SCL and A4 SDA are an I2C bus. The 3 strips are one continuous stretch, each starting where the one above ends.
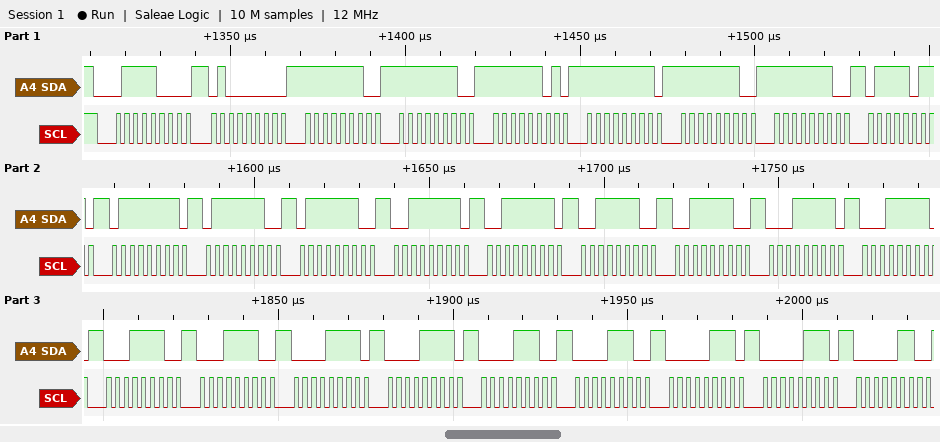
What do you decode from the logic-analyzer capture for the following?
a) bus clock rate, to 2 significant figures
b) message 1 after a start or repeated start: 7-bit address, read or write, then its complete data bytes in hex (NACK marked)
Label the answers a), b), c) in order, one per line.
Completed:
a) 400 kHz
b) 0x3C write: 40 FE FE FD FF FE FE 7B 7F 7E 7E 3F 3F 3E 3E 1F 1F 1E 1E 0F 0F 0E 0E 07 07 06
